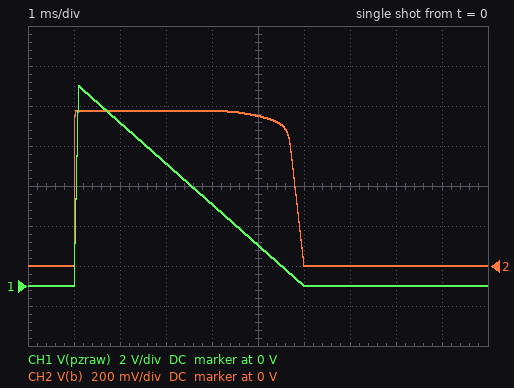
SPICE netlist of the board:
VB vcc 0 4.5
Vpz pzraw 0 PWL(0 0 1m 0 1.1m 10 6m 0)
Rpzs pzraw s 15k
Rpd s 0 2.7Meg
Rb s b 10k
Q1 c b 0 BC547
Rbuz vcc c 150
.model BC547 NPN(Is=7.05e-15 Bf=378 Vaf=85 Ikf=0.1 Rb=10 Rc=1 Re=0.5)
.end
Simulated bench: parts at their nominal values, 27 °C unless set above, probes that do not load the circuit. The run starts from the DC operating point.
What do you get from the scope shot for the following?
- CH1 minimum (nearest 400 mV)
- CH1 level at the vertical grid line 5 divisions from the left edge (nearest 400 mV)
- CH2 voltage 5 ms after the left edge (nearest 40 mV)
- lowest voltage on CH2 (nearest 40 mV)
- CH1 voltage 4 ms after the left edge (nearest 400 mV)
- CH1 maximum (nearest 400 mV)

0 V
2.0 V
760 mV
0 V
4.0 V
10.0 V
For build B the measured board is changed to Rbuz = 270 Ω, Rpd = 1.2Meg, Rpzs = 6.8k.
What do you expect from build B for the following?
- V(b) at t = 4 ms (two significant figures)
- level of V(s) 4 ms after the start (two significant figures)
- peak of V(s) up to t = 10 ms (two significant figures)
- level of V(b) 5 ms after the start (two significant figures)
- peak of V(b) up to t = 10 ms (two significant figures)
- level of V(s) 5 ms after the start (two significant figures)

750 mV
2.7 V
6.2 V
750 mV
760 mV
1.5 V
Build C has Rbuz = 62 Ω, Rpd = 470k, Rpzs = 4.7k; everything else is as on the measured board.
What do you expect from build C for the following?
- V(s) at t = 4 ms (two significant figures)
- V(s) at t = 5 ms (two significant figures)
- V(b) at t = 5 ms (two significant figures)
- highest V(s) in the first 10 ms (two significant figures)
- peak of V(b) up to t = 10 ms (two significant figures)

3.0 V
1.6 V
770 mV
7.0 V
830 mV
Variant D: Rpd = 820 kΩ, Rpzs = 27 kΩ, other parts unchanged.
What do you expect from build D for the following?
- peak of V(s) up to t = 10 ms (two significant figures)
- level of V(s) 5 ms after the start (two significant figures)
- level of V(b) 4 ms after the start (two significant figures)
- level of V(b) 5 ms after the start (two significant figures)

3.2 V
1.1 V
770 mV
740 mV
